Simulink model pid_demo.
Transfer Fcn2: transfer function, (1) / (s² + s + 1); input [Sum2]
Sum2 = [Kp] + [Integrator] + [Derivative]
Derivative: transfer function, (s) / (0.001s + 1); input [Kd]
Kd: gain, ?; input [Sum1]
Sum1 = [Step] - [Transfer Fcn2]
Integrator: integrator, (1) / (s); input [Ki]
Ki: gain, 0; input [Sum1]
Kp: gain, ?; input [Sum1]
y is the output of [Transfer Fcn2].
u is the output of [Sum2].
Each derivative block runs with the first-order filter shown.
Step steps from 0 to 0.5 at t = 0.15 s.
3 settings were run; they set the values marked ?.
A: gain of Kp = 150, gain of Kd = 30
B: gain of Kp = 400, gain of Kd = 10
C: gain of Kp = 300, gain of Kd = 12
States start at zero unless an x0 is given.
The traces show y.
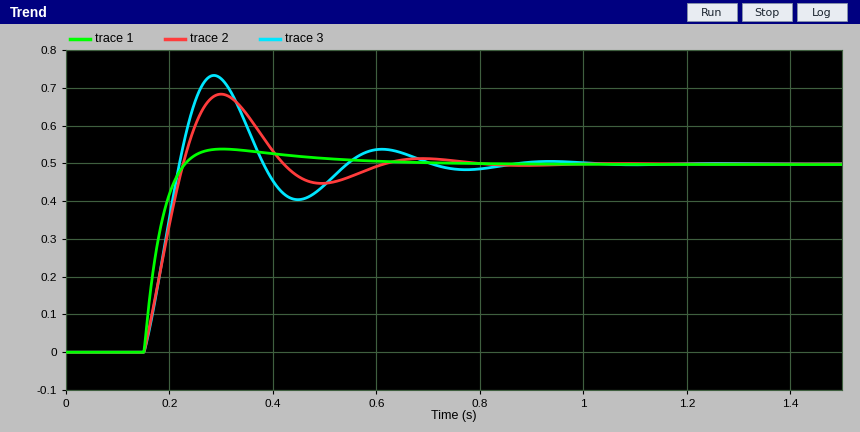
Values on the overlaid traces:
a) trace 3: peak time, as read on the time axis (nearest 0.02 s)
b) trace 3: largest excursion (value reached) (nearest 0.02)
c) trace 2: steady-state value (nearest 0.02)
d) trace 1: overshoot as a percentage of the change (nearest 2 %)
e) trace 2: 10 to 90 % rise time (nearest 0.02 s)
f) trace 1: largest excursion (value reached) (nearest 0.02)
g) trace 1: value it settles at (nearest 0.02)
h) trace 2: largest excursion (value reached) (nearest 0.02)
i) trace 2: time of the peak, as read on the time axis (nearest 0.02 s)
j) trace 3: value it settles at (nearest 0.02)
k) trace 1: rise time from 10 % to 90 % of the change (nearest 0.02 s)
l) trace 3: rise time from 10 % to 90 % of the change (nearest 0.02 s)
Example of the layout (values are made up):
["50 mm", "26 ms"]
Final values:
["0.28 s", "0.74", "0.50", "8 %", "0.06 s", "0.54", "0.50", "0.68", "0.30 s", "0.50", "0.06 s", "0.06 s"]
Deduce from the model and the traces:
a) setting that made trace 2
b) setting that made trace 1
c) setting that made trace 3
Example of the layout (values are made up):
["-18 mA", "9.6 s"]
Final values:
["C", "A", "B"]
